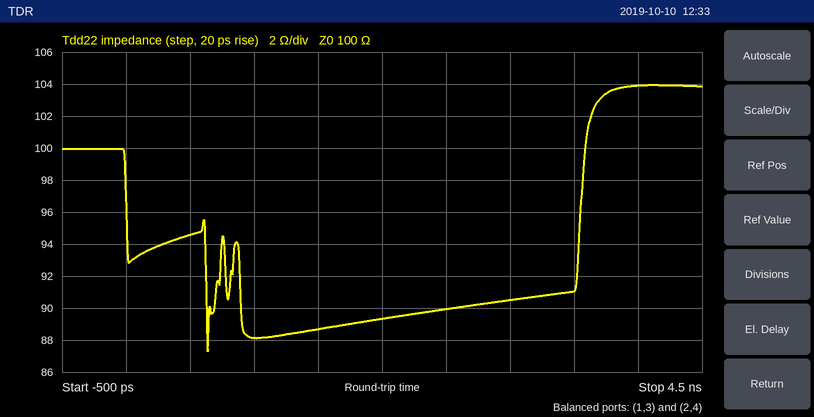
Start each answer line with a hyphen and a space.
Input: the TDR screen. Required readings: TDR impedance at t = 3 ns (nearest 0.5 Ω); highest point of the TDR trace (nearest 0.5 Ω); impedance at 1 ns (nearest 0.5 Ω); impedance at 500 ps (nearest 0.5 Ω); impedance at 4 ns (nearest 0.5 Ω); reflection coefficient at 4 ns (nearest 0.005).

- 90.5 Ω
- 104.0 Ω
- 88.0 Ω
- 94.5 Ω
- 104.0 Ω
- +0.020
